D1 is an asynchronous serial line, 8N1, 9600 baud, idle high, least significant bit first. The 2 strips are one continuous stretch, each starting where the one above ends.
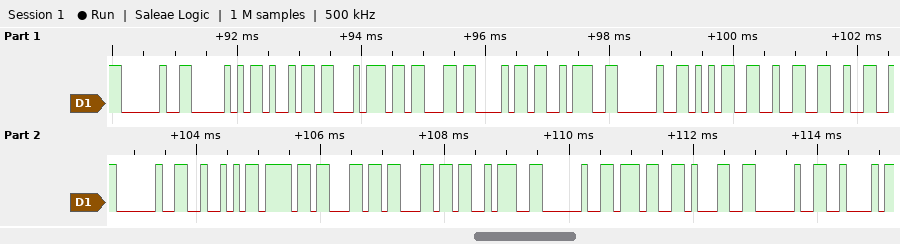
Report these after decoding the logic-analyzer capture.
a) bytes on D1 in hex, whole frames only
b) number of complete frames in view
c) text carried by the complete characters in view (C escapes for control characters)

20 50 69 74 63 68 3A 20 35 32 32 20 52 6F 6C 6C 3A 20 37 31 20 42
22
" Pitch: 522 Roll: 71 B"
